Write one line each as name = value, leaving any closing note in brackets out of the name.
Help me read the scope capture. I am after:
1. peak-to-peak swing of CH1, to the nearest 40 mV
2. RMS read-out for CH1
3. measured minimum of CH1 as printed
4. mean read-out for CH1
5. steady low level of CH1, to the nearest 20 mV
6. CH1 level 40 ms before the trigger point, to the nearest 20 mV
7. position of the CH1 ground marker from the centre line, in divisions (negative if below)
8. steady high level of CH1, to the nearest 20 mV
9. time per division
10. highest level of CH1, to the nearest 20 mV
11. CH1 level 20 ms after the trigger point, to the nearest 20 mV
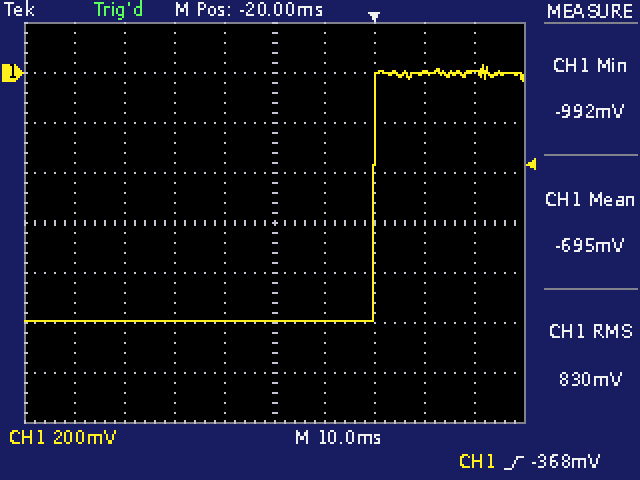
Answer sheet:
peak-to-peak swing of CH1, to the nearest 40 mV = 1.04 V
RMS read-out for CH1 = 830 mV
measured minimum of CH1 as printed = -992 mV
mean read-out for CH1 = -695 mV
steady low level of CH1, to the nearest 20 mV = -1.00 V
CH1 level 40 ms before the trigger point, to the nearest 20 mV = -1.00 V
position of the CH1 ground marker from the centre line, in divisions = +3.0 div
steady high level of CH1, to the nearest 20 mV = 0 mV
time per division = 10 ms
highest level of CH1, to the nearest 20 mV = 40 mV
CH1 level 20 ms after the trigger point, to the nearest 20 mV = 0 mV
